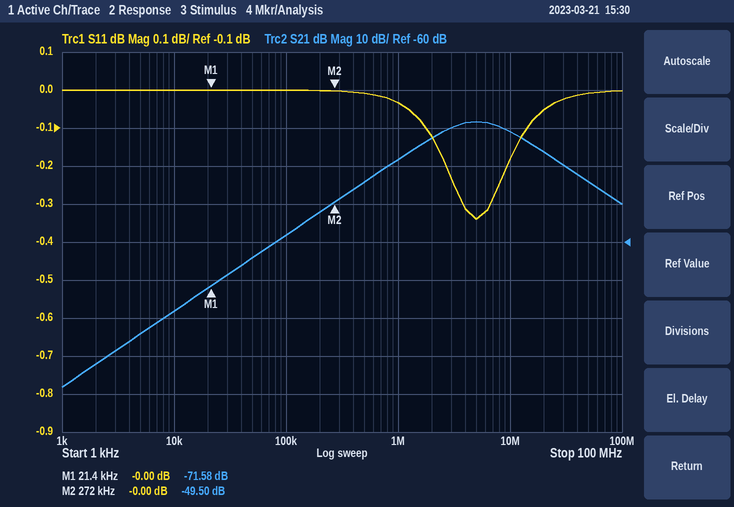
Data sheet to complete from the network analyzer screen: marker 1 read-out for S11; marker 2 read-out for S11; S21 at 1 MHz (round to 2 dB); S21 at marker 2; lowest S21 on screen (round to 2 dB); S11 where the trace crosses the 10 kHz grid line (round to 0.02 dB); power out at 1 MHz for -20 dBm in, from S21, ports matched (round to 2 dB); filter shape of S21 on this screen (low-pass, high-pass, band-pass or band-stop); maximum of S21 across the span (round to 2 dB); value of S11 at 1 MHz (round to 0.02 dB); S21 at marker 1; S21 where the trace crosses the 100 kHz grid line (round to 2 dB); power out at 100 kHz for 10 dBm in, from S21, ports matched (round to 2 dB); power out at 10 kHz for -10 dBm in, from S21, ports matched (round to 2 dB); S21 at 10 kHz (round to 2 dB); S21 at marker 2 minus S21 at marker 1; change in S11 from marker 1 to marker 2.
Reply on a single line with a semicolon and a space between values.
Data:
-0.00 dB; -0.00 dB; -38 dB; -49.50 dB; -98 dB; 0.00 dB; -58 dBm; band-pass; -28 dB; -0.04 dB; -71.58 dB; -58 dB; -48 dBm; -88 dBm; -78 dB; 22.08 dB; 0.00 dB
